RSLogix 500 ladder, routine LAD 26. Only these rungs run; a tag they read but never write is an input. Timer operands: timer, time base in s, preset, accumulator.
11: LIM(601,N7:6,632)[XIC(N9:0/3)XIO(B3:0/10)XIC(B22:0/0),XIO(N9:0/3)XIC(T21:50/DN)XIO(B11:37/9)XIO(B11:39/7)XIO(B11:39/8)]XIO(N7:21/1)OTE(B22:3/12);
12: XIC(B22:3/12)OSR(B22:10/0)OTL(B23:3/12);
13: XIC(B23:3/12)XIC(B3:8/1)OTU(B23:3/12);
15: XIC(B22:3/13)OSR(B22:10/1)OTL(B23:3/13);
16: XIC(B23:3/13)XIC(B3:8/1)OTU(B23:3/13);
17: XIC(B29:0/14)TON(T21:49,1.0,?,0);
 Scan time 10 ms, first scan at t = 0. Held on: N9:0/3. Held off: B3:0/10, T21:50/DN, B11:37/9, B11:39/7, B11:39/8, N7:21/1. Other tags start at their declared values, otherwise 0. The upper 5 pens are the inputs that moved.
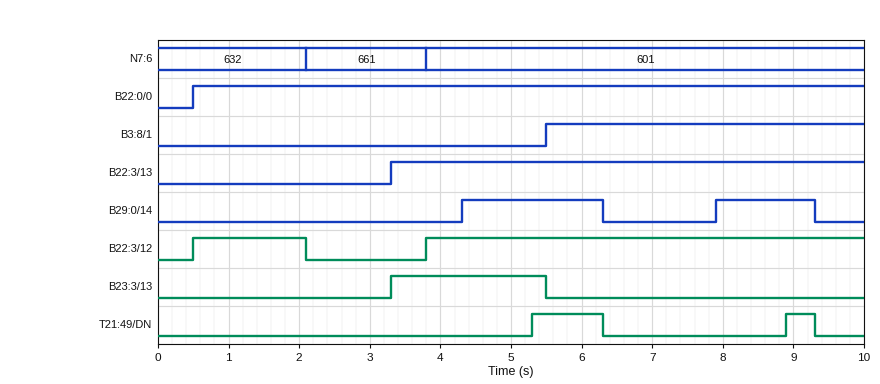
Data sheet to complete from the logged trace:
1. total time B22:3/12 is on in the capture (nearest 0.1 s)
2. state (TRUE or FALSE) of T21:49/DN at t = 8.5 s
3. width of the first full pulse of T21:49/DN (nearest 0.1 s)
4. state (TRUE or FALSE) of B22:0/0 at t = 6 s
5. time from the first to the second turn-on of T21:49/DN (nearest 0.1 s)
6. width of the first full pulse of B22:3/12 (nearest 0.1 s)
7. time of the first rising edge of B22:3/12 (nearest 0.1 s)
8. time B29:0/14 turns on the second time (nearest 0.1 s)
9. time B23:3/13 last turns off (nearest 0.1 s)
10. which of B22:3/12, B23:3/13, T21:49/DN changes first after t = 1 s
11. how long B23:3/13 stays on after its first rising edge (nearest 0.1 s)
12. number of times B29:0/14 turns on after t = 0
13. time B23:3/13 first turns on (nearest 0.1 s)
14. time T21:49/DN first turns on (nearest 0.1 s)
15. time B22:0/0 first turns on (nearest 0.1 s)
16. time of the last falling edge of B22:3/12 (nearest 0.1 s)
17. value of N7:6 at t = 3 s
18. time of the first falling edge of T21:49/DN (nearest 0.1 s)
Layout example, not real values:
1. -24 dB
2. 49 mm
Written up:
1. 7.8 s
2. FALSE
3. 1.0 s
4. TRUE
5. 3.6 s
6. 1.6 s
7. 0.5 s
8. 7.9 s
9. 5.5 s
10. B22:3/12
11. 2.2 s
12. 2
13. 3.3 s
14. 5.3 s
15. 0.5 s
16. 2.1 s
17. 661
18. 6.3 s
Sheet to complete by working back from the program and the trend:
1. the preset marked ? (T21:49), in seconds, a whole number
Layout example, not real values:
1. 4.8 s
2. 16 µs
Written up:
1. 1 s
